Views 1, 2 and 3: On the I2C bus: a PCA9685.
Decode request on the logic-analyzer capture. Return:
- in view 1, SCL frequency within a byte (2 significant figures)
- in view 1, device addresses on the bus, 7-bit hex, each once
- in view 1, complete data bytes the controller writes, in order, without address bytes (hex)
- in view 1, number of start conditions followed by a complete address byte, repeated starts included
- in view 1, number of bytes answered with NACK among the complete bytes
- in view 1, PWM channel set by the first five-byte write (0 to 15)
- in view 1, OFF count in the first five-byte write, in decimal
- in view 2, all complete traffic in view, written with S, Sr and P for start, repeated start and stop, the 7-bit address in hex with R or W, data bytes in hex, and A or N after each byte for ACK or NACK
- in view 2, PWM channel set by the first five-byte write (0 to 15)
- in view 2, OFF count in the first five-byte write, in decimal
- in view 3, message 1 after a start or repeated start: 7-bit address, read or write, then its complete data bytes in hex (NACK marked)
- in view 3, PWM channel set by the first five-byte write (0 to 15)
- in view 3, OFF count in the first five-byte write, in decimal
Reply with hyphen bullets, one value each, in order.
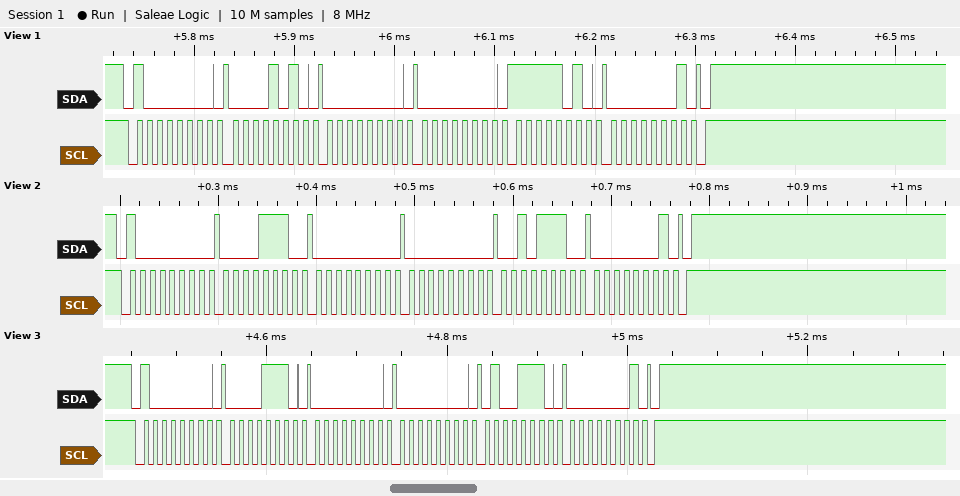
- 100 kHz
- 0x40
- 0A 00 00 FA 01
- 1
- 0
- 1
- 506
- S 40W A 0E A 00 A 00 A 2E A 01 A P
- 2
- 302
- 0x40 write: 0E 00 00 4E 01
- 2
- 334
